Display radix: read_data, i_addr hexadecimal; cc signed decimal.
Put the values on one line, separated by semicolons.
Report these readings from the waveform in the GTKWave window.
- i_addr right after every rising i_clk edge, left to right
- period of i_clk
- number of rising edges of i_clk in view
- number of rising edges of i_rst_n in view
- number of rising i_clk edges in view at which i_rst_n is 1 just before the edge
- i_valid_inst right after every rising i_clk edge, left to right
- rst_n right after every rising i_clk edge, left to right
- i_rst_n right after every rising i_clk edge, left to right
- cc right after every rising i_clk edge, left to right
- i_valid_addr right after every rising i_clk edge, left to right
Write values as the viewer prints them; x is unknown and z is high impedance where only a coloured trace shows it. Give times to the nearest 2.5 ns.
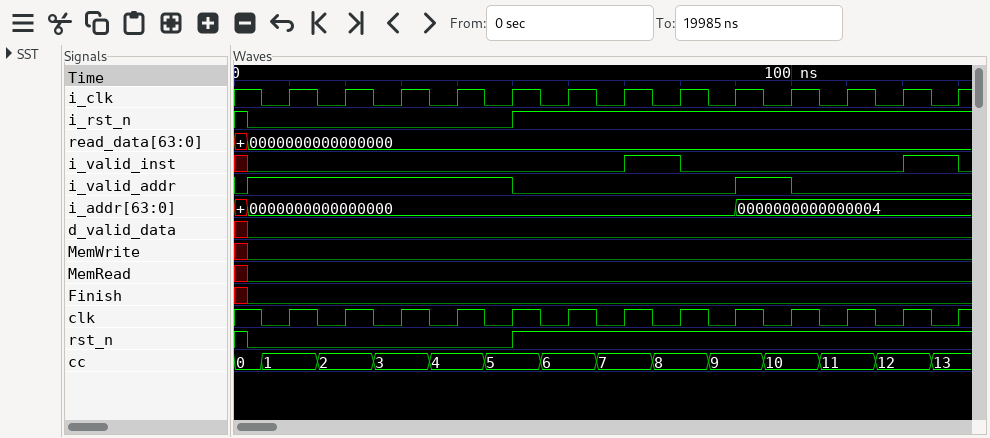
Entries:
0000000000000000, 0000000000000000, 0000000000000000, 0000000000000000, 0000000000000000, 0000000000000000, 0000000000000000, 0000000000000000, 0000000000000004, 0000000000000004, 0000000000000004, 0000000000000004, 0000000000000004; 10 ns; 13; 1; 8; 0 0 0 0 0 0 1 0 0 0 0 1 0; 0 0 0 0 1 1 1 1 1 1 1 1 1; 0 0 0 0 1 1 1 1 1 1 1 1 1; 1, 2, 3, 4, 5, 6, 7, 8, 9, 10, 11, 12, 13; 1 1 1 1 0 0 0 0 1 0 0 0 0
